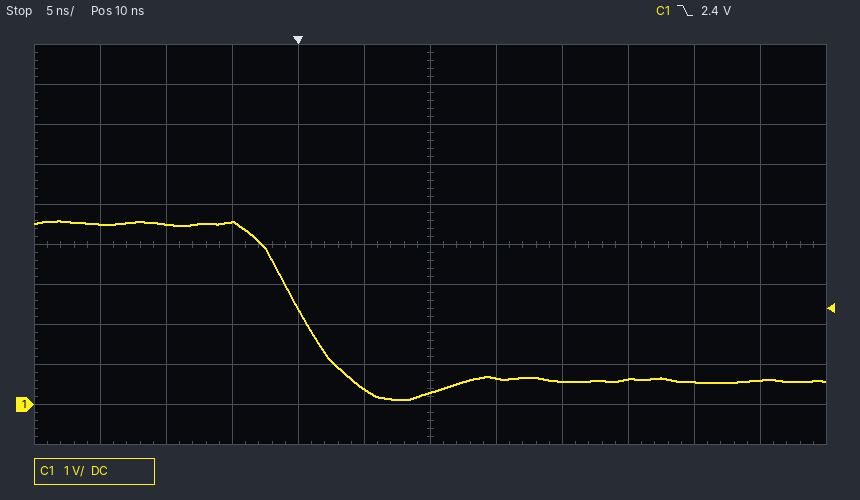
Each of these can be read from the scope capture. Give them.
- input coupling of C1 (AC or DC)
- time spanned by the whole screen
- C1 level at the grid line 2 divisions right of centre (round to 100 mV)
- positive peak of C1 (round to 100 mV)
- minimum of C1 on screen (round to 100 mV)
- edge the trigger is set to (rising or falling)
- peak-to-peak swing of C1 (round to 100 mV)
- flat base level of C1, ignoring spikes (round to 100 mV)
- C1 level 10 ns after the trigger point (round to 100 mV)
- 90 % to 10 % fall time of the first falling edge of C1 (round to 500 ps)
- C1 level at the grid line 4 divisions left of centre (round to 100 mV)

DC
60 ns
600 mV
4.6 V
100 mV
falling
4.5 V
600 mV
300 mV
6.0 ns
4.5 V
